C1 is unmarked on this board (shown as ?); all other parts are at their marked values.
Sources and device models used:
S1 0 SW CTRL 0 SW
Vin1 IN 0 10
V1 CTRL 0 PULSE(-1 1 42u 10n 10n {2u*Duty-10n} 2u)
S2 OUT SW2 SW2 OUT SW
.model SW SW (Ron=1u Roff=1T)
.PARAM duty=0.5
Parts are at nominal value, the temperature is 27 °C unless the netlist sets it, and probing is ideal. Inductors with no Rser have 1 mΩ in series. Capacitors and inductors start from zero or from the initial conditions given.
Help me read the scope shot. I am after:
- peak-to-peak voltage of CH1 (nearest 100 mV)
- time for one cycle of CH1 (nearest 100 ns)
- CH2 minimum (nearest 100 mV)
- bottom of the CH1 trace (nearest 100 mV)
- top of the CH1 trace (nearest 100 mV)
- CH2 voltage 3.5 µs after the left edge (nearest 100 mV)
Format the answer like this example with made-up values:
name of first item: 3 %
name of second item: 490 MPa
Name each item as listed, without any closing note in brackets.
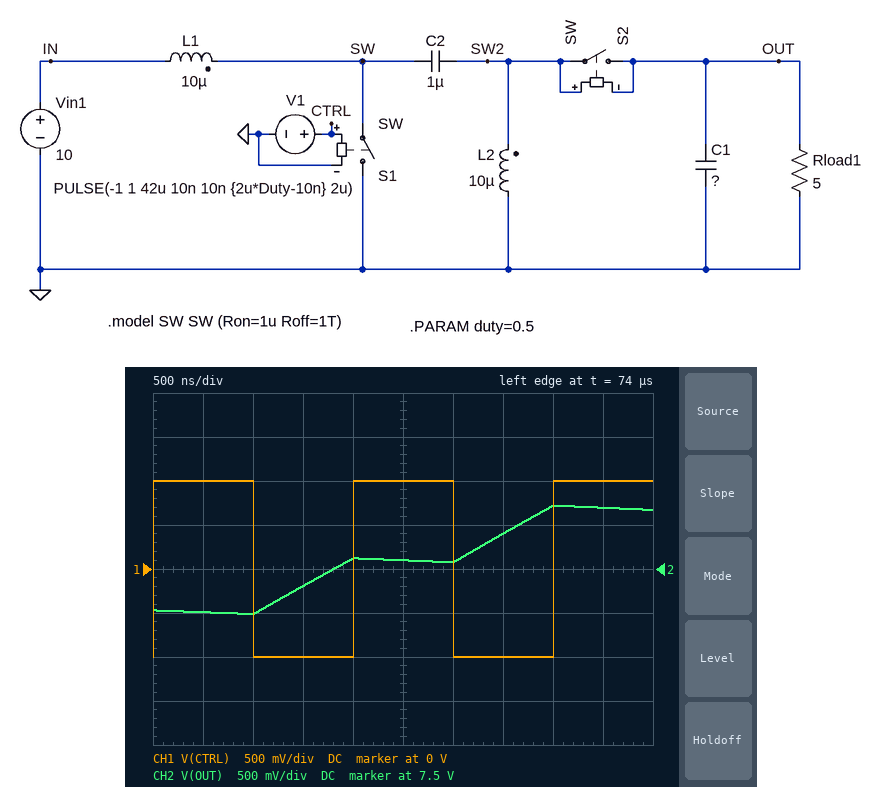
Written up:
peak-to-peak voltage of CH1: 2.0 V
time for one cycle of CH1: 2.0 µs
CH2 minimum: 7.0 V
bottom of the CH1 trace: -1.0 V
top of the CH1 trace: 1.0 V
CH2 voltage 3.5 µs after the left edge: 7.9 V
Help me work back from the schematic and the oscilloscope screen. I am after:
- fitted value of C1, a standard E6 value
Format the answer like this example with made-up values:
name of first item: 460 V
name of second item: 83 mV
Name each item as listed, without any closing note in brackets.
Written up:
fitted value of C1, a standard E6 value: 33 µF
